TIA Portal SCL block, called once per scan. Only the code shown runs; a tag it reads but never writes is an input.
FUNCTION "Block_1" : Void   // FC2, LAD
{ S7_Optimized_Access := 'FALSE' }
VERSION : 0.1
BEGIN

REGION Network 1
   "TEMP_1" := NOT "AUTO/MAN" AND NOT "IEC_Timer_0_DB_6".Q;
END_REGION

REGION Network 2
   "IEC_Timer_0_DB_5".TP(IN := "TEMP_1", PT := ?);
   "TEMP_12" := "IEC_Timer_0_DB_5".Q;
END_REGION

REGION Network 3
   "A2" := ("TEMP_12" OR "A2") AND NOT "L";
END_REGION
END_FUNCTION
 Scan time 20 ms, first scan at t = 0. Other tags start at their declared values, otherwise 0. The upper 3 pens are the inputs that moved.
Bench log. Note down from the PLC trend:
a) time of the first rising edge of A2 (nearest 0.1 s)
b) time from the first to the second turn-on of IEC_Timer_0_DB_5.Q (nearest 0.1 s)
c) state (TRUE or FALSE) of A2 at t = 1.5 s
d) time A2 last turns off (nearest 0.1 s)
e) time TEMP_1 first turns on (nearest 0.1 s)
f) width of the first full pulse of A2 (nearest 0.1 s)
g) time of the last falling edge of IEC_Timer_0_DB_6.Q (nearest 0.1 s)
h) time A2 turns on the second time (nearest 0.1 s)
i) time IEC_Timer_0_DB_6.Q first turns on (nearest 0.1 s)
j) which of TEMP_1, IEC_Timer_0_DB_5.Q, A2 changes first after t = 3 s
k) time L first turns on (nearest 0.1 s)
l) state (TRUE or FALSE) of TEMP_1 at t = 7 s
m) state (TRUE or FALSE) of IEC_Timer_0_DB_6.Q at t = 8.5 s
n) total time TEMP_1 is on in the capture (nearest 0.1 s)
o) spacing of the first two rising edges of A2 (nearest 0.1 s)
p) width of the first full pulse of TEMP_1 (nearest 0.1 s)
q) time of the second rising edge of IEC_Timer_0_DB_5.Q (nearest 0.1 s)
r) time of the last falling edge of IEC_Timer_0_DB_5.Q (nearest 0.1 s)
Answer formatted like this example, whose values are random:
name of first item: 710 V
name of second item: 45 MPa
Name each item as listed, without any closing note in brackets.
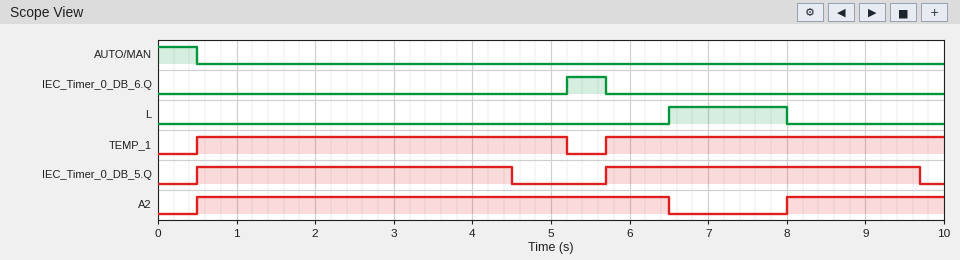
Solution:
time of the first rising edge of A2: 0.5 s
time from the first to the second turn-on of IEC_Timer_0_DB_5.Q: 5.2 s
state (TRUE or FALSE) of A2 at t = 1.5 s: TRUE
time A2 last turns off: 6.5 s
time TEMP_1 first turns on: 0.5 s
width of the first full pulse of A2: 6.0 s
time of the last falling edge of IEC_Timer_0_DB_6.Q: 5.7 s
time A2 turns on the second time: 8.0 s
time IEC_Timer_0_DB_6.Q first turns on: 5.2 s
which of TEMP_1, IEC_Timer_0_DB_5.Q, A2 changes first after t = 3 s: IEC_Timer_0_DB_5.Q
time L first turns on: 6.5 s
state (TRUE or FALSE) of TEMP_1 at t = 7 s: TRUE
state (TRUE or FALSE) of IEC_Timer_0_DB_6.Q at t = 8.5 s: FALSE
total time TEMP_1 is on in the capture: 9.0 s
spacing of the first two rising edges of A2: 7.5 s
width of the first full pulse of TEMP_1: 4.7 s
time of the second rising edge of IEC_Timer_0_DB_5.Q: 5.7 s
time of the last falling edge of IEC_Timer_0_DB_5.Q: 9.7 s
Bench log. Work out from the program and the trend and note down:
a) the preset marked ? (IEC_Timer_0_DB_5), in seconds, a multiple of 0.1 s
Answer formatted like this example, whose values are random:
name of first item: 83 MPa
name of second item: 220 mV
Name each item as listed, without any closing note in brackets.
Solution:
the preset marked ? (IEC_Timer_0_DB_5), in seconds, a multiple of 0.1 s: 4.0 s
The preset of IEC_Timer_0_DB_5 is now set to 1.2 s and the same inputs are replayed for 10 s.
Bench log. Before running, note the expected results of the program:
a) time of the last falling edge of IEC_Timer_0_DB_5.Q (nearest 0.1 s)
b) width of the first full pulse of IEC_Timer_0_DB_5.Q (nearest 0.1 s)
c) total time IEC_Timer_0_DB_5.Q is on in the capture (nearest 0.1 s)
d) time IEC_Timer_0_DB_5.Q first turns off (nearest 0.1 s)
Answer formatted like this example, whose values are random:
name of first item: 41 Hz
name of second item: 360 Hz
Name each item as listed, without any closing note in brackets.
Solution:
time of the last falling edge of IEC_Timer_0_DB_5.Q: 6.9 s
width of the first full pulse of IEC_Timer_0_DB_5.Q: 1.2 s
total time IEC_Timer_0_DB_5.Q is on in the capture: 2.4 s
time IEC_Timer_0_DB_5.Q first turns off: 1.7 s
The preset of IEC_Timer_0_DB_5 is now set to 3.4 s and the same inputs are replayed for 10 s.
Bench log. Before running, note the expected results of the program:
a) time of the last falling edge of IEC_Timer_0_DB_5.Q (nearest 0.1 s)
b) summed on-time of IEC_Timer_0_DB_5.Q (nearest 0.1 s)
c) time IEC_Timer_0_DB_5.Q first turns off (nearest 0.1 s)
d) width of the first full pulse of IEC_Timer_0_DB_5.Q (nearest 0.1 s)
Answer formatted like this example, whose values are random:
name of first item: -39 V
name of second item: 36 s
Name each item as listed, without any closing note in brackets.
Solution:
time of the last falling edge of IEC_Timer_0_DB_5.Q: 9.1 s
summed on-time of IEC_Timer_0_DB_5.Q: 6.8 s
time IEC_Timer_0_DB_5.Q first turns off: 3.9 s
width of the first full pulse of IEC_Timer_0_DB_5.Q: 3.4 s
